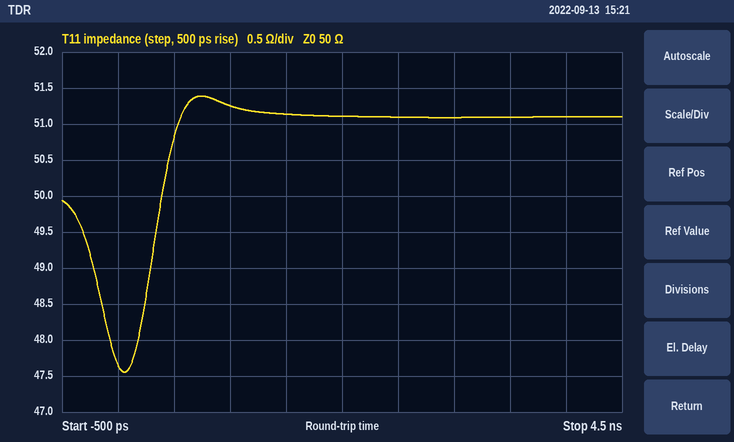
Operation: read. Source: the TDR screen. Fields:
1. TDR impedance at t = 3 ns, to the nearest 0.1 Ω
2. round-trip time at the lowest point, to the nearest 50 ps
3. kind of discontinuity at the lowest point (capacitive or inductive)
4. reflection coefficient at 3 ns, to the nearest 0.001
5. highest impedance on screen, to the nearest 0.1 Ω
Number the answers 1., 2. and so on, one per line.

1. 51.1 Ω
2. 50 ps
3. capacitive
4. +0.011
5. 51.4 Ω
